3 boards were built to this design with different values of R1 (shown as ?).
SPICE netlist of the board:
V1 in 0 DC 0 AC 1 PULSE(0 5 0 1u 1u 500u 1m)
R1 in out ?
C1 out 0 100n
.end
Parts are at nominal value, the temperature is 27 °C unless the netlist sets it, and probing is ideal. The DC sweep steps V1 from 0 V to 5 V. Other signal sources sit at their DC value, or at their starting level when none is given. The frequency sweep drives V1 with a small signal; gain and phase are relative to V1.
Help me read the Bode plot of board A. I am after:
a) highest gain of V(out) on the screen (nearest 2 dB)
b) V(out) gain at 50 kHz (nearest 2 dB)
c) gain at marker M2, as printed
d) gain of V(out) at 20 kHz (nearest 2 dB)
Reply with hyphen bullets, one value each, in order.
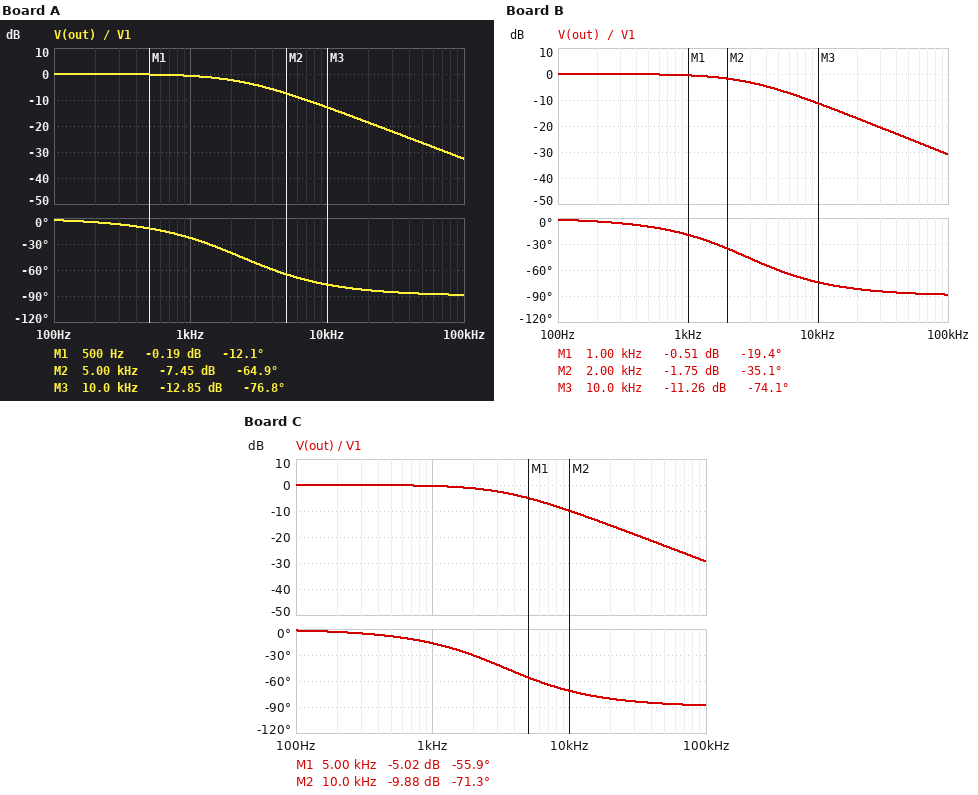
- 0 dB
- -26 dB
- -7.45 dB
- -18 dB
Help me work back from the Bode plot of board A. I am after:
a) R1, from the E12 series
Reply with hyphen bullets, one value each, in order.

- 680 Ω
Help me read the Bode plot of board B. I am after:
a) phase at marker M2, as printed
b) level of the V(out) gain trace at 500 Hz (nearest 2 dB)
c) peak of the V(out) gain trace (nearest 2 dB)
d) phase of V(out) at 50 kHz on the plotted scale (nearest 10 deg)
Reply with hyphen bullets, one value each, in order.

- -35.1 deg
- 0 dB
- 0 dB
- -90 deg
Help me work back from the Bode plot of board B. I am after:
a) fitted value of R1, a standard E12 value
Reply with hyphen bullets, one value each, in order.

- 560 Ω
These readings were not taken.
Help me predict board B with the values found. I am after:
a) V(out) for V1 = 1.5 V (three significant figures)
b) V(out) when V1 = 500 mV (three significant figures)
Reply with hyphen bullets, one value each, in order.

- 1.50 V
- 500 mV
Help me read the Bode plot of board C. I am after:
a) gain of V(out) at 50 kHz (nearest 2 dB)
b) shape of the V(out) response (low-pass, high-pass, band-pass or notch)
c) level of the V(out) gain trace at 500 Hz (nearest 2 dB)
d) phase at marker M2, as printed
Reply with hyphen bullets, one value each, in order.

- -24 dB
- low-pass
- 0 dB
- -71.3 deg
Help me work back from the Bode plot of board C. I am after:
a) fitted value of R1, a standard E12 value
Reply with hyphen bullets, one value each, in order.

- 470 Ω
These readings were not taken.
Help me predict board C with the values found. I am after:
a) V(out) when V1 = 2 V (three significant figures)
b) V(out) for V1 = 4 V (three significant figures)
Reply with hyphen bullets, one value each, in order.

- 2.00 V
- 4.00 V
